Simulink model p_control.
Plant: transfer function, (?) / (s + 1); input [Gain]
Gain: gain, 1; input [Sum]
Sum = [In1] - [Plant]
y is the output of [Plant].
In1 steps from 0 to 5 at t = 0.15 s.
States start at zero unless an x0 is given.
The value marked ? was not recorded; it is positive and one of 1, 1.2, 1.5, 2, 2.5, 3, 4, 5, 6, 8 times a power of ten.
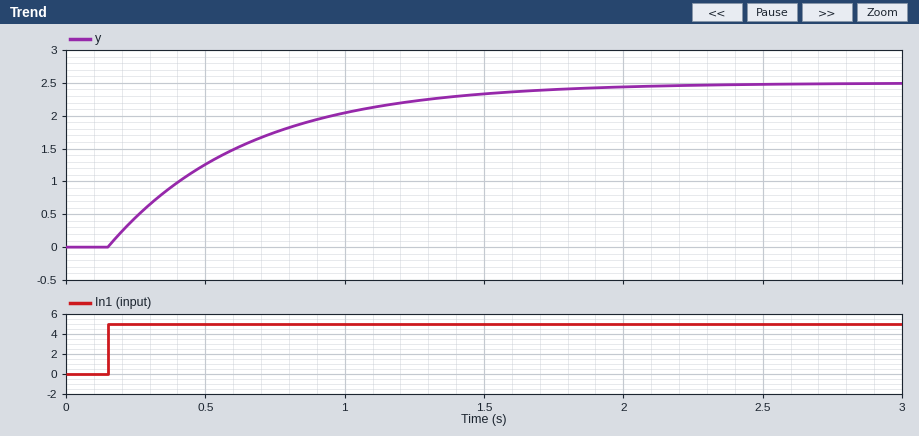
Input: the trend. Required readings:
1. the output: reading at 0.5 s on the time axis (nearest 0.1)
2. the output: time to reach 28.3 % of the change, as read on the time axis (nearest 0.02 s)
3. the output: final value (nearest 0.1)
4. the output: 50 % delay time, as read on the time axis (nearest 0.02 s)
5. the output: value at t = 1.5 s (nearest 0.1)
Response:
1.3
0.32 s
2.5
0.50 s
2.3
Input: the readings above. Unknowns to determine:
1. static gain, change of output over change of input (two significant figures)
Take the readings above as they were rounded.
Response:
0.50
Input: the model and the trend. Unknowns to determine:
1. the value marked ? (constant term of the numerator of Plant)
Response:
1
